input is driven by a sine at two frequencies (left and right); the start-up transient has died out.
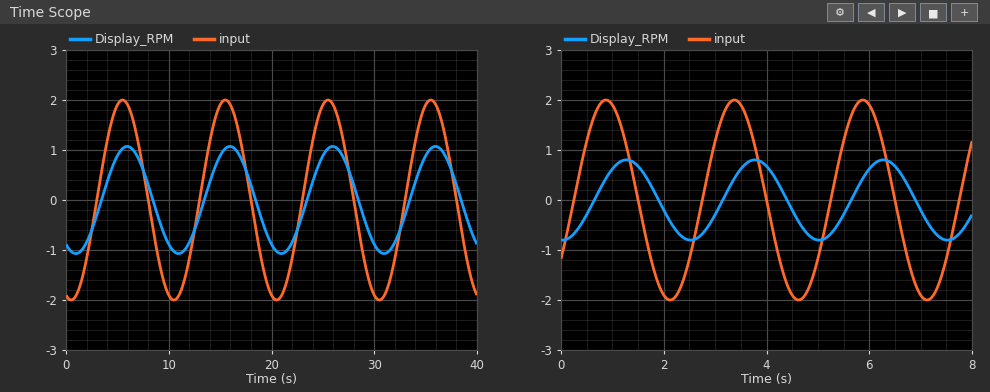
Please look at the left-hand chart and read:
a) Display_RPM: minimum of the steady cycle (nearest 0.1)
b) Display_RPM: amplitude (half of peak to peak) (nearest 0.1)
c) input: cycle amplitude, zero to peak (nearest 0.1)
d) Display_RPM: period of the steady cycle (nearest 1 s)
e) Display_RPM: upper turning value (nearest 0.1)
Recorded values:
-1.1
1.1
2.0
10 s
1.1
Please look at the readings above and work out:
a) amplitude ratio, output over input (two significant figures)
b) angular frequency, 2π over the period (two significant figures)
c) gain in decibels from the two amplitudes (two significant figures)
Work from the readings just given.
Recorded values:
0.55
0.63 rad/s
-5.2 dB
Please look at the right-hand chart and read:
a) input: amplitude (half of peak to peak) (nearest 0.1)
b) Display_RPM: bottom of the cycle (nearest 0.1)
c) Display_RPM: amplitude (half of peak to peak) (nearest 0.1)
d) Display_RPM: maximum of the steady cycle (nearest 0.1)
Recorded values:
2.0
-0.8
0.8
0.8
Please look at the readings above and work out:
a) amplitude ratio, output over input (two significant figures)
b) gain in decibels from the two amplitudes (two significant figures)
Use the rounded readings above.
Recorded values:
0.40
-8.0 dB
